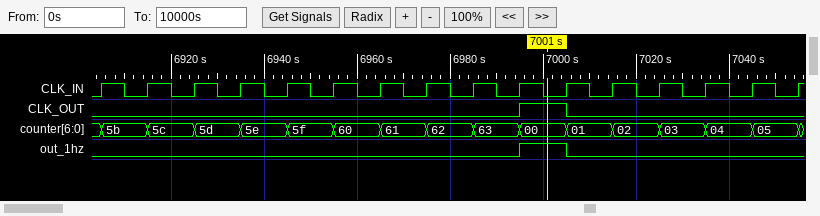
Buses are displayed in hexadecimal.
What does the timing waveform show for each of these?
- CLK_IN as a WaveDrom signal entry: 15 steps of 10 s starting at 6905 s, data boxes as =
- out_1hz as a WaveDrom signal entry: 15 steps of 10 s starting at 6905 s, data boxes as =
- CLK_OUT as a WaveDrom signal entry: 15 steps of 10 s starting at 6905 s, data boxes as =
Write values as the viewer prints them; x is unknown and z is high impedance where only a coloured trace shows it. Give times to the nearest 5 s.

{name: 'CLK_IN', wave: 'p..............'}
{name: 'out_1hz', wave: '0........10....'}
{name: 'CLK_OUT', wave: '0........10....'}
